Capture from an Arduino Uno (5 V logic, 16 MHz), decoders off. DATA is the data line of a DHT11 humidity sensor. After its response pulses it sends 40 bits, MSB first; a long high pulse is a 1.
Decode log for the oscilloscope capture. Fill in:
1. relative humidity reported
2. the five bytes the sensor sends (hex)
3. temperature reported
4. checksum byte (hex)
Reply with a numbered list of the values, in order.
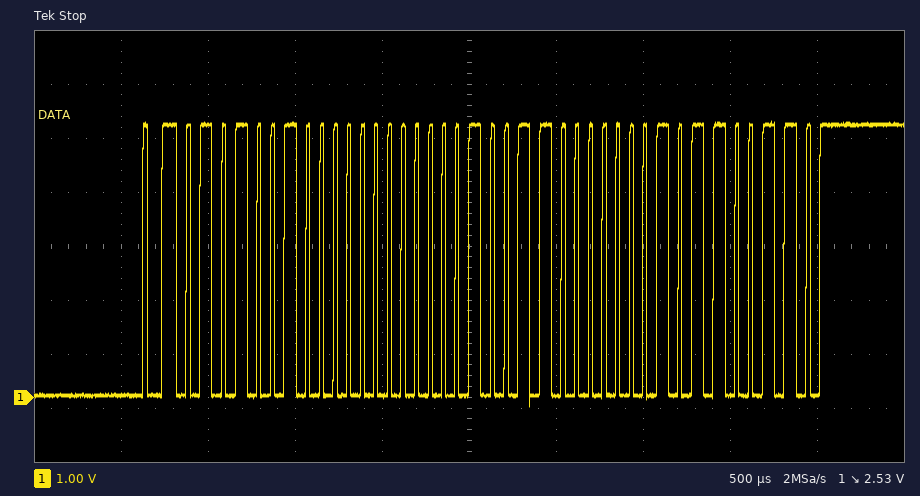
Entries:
1. 82 %
2. 52 00 13 01 66
3. 19.1 °C
4. 0x66
